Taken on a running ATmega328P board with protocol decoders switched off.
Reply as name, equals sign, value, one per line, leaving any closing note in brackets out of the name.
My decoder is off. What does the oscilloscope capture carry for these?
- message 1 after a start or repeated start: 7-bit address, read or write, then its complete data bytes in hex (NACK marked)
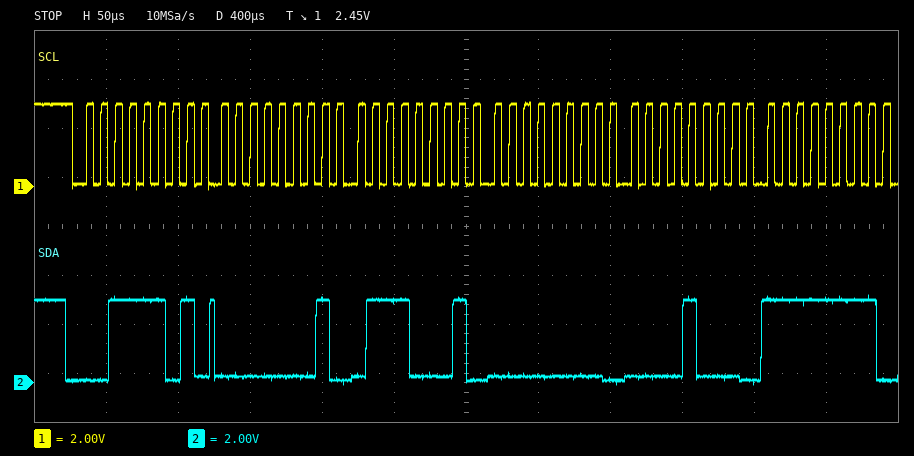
message 1 after a start or repeated start: 7-bit address, read or write, then its complete data bytes in hex = 0x1E read: 01 71 00 08 FF
